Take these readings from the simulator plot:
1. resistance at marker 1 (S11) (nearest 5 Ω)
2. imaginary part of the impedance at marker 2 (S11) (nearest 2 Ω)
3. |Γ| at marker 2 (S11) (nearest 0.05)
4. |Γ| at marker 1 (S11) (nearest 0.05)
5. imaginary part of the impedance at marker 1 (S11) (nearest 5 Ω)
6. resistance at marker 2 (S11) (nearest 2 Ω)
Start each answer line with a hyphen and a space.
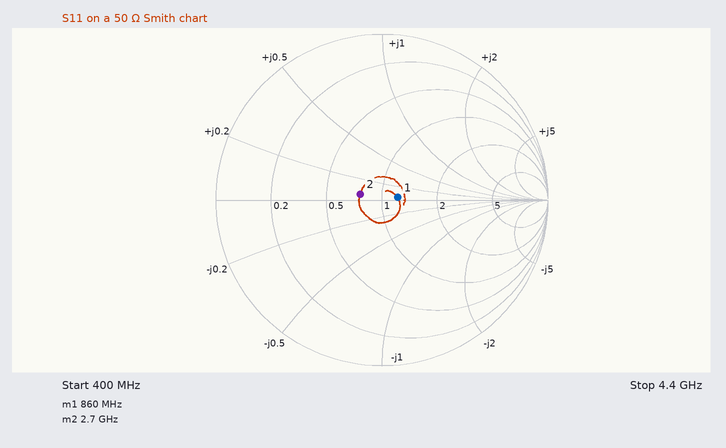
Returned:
- 60 Ω
- +2 Ω
- 0.15
- 0.10
- 0 Ω
- 38 Ω
